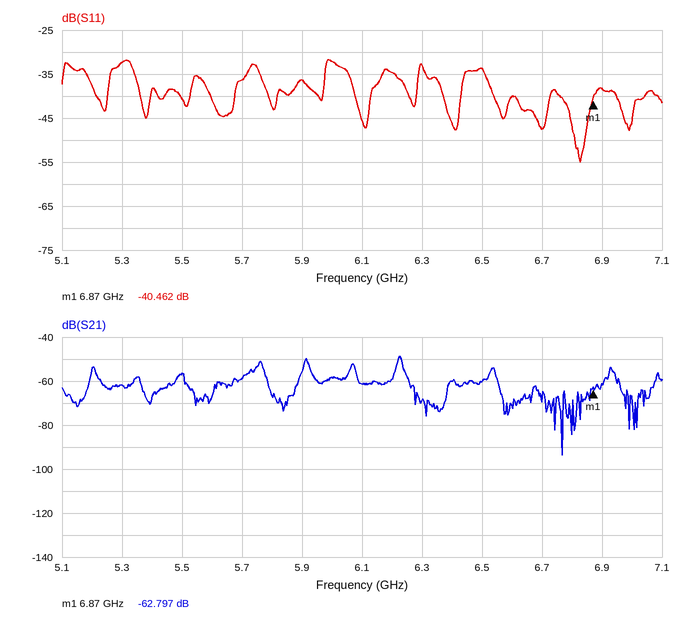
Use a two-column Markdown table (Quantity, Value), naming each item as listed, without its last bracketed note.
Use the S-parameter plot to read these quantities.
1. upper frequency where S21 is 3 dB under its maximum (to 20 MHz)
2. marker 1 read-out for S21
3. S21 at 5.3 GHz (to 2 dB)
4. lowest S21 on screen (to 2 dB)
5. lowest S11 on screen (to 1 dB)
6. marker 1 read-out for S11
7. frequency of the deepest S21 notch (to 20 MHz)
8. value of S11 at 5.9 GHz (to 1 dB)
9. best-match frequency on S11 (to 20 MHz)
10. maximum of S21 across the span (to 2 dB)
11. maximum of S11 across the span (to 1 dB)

| Quantity | Value |
|---|---|
| upper frequency where S21 is 3 dB under its maximum | 6.24 GHz |
| marker 1 read-out for S21 | -62.797 dB |
| S21 at 5.3 GHz | -62 dB |
| lowest S21 on screen | -94 dB |
| lowest S11 on screen | -55 dB |
| marker 1 read-out for S11 | -40.462 dB |
| frequency of the deepest S21 notch | 6.76 GHz |
| value of S11 at 5.9 GHz | -36 dB |
| best-match frequency on S11 | 6.82 GHz |
| maximum of S21 across the span | -48 dB |
| maximum of S11 across the span | -32 dB |
